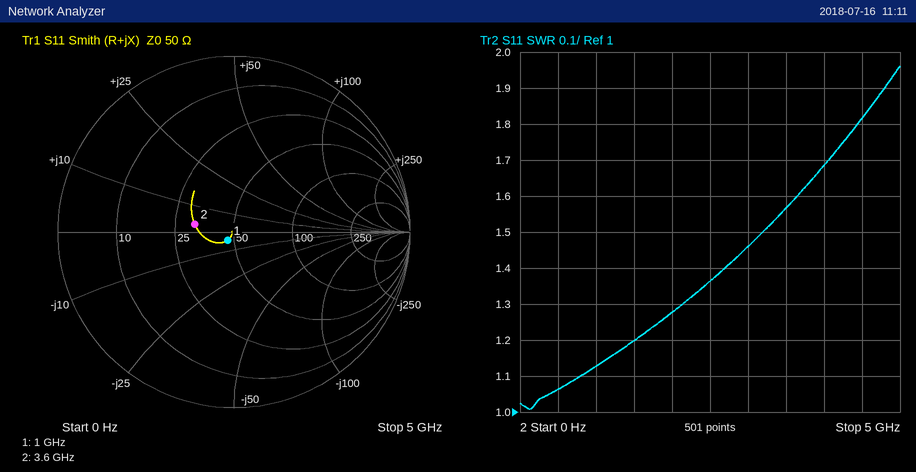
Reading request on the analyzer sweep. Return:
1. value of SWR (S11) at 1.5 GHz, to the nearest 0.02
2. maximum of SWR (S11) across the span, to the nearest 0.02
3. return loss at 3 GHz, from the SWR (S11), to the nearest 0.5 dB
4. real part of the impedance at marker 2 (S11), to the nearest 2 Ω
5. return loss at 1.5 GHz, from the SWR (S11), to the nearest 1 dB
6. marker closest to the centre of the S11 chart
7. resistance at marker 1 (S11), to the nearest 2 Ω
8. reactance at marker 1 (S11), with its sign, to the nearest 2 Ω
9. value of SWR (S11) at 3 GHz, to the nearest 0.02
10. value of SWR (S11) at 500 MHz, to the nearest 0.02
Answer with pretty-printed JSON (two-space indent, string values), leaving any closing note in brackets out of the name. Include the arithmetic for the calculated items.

{
  "value of SWR (S11) at 1.5 GHz, to the nearest 0.02": "1.20",
  "maximum of SWR (S11) across the span, to the nearest 0.02": "1.96",
  "return loss at 3 GHz, from the SWR (S11), to the nearest 0.5 dB": "−20 log10((1.46 − 1)/(1.46 + 1)) ≈ 14.6 dB, so 14.5 dB to the nearest 0.5 dB",
  "real part of the impedance at marker 2 (S11), to the nearest 2 Ω": "32 Ω",
  "return loss at 1.5 GHz, from the SWR (S11), to the nearest 1 dB": "−20 log10((1.2 − 1)/(1.2 + 1)) ≈ 21 dB",
  "marker closest to the centre of the S11 chart": "marker 1",
  "resistance at marker 1 (S11), to the nearest 2 Ω": "46 Ω",
  "reactance at marker 1 (S11), with its sign, to the nearest 2 Ω": "-4 Ω",
  "value of SWR (S11) at 3 GHz, to the nearest 0.02": "1.46",
  "value of SWR (S11) at 500 MHz, to the nearest 0.02": "1.06"
}
